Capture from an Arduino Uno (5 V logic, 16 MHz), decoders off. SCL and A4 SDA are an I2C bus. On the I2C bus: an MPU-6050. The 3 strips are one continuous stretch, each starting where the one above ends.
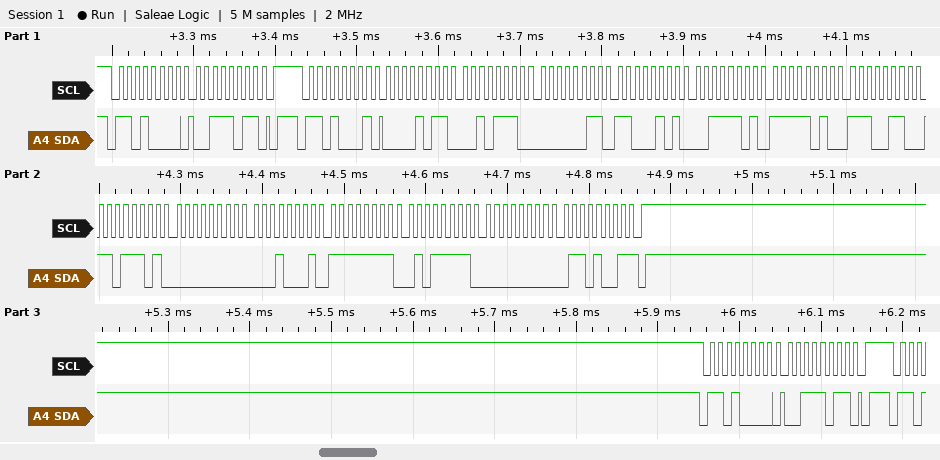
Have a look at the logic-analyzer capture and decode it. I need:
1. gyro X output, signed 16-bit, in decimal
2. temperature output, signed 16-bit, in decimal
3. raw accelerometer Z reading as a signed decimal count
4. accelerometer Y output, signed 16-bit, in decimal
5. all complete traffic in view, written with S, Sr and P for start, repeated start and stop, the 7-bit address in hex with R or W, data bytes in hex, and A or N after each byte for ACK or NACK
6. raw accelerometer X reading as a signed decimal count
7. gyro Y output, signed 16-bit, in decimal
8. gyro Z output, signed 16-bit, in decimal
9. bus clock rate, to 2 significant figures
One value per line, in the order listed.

17
-6435
15866
965
S 68W A 3B A P S 68R A 0B A 2E A 03 A C5 A 3D A FA A E6 A DD A 00 A 11 A FF A 5F A 00 A 69 N P S 68W A 3B A P
2862
-161
105
100 kHz
